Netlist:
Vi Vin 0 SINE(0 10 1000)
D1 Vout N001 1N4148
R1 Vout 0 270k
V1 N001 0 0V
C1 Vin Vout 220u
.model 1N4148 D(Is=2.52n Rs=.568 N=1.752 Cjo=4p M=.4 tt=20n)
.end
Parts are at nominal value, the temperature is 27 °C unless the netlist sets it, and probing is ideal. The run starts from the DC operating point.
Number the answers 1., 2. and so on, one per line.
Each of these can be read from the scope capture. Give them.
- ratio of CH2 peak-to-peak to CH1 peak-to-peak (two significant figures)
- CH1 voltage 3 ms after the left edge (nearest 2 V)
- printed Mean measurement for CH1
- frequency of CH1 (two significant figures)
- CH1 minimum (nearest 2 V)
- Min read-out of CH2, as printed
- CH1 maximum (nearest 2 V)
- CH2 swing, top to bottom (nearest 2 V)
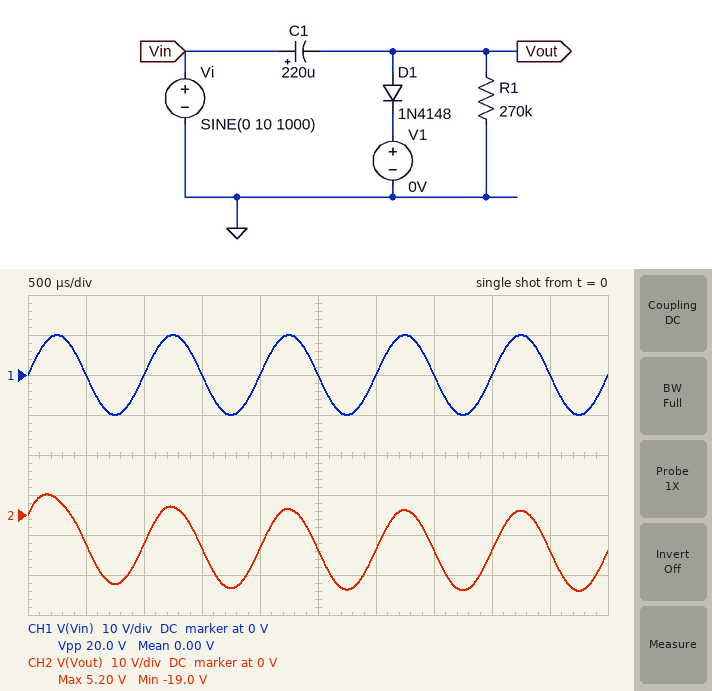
1. 1.2
2. 0 V
3. 0.00 V
4. 1.0 kHz
5. -10 V
6. -19.0 V
7. 10 V
8. 24 V
